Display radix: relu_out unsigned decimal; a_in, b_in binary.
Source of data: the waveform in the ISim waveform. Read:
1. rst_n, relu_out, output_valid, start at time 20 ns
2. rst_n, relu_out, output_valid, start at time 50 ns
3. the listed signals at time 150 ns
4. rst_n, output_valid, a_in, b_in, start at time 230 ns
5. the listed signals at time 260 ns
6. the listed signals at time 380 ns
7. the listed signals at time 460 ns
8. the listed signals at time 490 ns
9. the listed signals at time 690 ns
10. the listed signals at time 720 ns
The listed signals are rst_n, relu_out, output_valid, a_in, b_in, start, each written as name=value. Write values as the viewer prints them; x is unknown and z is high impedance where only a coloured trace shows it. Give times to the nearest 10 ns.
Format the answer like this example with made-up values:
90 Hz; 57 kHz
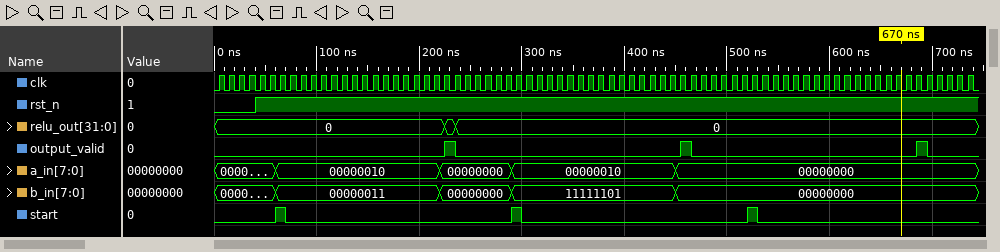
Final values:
rst_n=0, relu_out=0, output_valid=0, start=0; rst_n=1, relu_out=0, output_valid=0, start=0; rst_n=1, relu_out=0, output_valid=0, a_in=00000010, b_in=00000011, start=0; rst_n=1, output_valid=1, a_in=00000000, b_in=00000000, start=0; rst_n=1, relu_out=0, output_valid=0, a_in=00000000, b_in=00000000, start=0; rst_n=1, relu_out=0, output_valid=0, a_in=00000010, b_in=11111101, start=0; rst_n=1, relu_out=0, output_valid=1, a_in=00000000, b_in=00000000, start=0; rst_n=1, relu_out=0, output_valid=0, a_in=00000000, b_in=00000000, start=0; rst_n=1, relu_out=0, output_valid=1, a_in=00000000, b_in=00000000, start=0; rst_n=1, relu_out=0, output_valid=0, a_in=00000000, b_in=00000000, start=0
